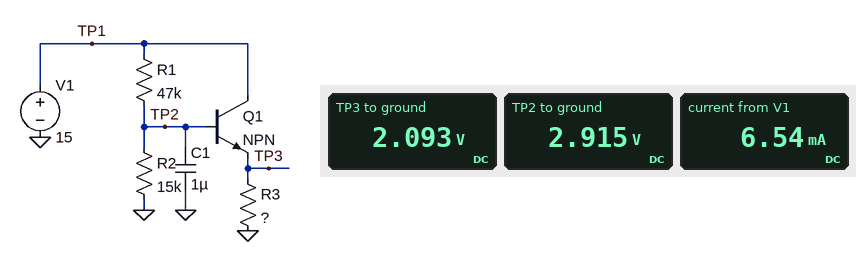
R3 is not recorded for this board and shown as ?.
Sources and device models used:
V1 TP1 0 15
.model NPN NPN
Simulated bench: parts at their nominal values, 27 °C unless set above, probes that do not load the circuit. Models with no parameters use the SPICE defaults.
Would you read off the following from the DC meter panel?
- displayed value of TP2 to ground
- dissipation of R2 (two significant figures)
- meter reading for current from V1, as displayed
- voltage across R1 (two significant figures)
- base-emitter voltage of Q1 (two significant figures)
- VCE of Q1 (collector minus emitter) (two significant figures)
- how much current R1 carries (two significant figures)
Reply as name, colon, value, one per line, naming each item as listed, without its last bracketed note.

displayed value of TP2 to ground: 2.915 V
dissipation of R2: 570 µW
meter reading for current from V1, as displayed: 6.54 mA
voltage across R1: 12 V
base-emitter voltage of Q1: 820 mV
VCE of Q1 (collector minus emitter): 13 V
how much current R1 carries: 260 µA
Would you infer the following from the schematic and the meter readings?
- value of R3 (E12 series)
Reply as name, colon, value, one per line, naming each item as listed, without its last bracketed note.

value of R3: 330 Ω
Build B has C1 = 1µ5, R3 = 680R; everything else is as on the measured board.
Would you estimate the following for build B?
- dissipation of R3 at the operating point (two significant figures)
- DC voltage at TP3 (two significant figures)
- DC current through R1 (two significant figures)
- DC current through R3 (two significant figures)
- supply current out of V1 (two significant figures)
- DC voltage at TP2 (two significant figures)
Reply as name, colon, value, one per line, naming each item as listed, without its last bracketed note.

dissipation of R3 at the operating point: 8.6 mW
DC voltage at TP3: 2.4 V
DC current through R1: 250 µA
DC current through R3: 3.6 mA
supply current out of V1: 3.8 mA
DC voltage at TP2: 3.2 V
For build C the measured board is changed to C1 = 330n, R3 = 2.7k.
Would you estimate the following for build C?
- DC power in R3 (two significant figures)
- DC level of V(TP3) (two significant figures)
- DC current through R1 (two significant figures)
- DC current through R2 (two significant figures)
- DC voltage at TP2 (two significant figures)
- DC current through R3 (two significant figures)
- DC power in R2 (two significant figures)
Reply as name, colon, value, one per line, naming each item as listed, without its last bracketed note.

DC power in R3: 2.8 mW
DC level of V(TP3): 2.7 V
DC current through R1: 240 µA
DC current through R2: 230 µA
DC voltage at TP2: 3.5 V
DC current through R3: 1.0 mA
DC power in R2: 820 µW
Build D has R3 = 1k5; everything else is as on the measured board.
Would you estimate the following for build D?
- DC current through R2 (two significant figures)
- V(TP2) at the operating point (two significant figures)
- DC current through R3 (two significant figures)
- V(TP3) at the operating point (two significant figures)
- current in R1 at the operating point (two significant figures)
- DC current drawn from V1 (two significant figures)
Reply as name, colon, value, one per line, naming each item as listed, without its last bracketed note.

DC current through R2: 230 µA
V(TP2) at the operating point: 3.4 V
DC current through R3: 1.8 mA
V(TP3) at the operating point: 2.6 V
current in R1 at the operating point: 250 µA
DC current drawn from V1: 2.0 mA
